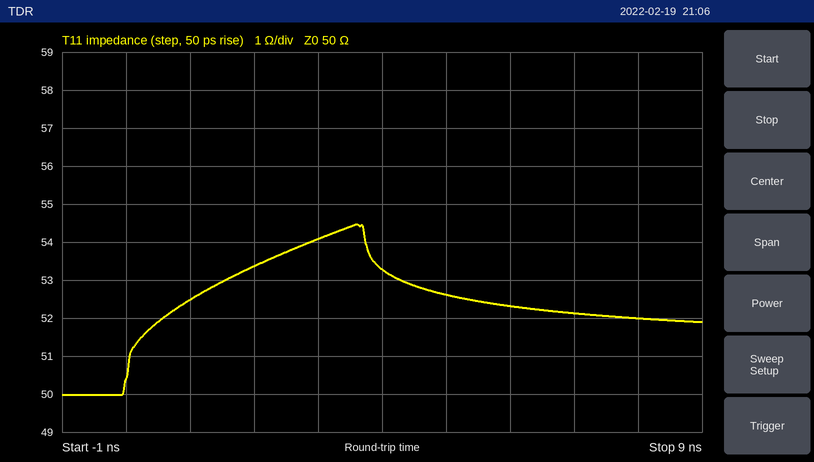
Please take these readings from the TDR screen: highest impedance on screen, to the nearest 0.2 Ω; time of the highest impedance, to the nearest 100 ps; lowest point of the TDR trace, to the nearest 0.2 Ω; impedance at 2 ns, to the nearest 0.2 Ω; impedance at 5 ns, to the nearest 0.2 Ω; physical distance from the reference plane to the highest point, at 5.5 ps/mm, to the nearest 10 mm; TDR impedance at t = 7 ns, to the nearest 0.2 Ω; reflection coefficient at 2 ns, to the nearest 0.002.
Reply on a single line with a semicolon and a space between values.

54.4 Ω; 3.6 ns; 50.0 Ω; 53.4 Ω; 52.6 Ω; 330 mm; 52.2 Ω; +0.032
